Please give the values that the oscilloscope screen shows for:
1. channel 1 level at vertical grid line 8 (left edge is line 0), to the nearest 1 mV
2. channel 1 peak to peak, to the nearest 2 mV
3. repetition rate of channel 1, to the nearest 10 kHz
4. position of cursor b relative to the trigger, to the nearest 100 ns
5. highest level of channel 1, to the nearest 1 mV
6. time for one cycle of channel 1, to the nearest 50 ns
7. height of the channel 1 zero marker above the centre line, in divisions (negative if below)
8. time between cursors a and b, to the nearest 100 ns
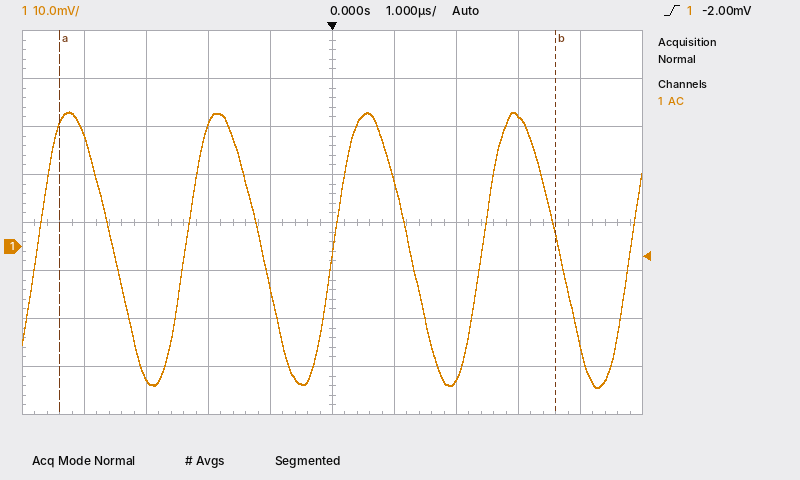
27 mV
58 mV
420 kHz
+3.6 µs
28 mV
2.40 µs
-0.5 div
8.0 µs
